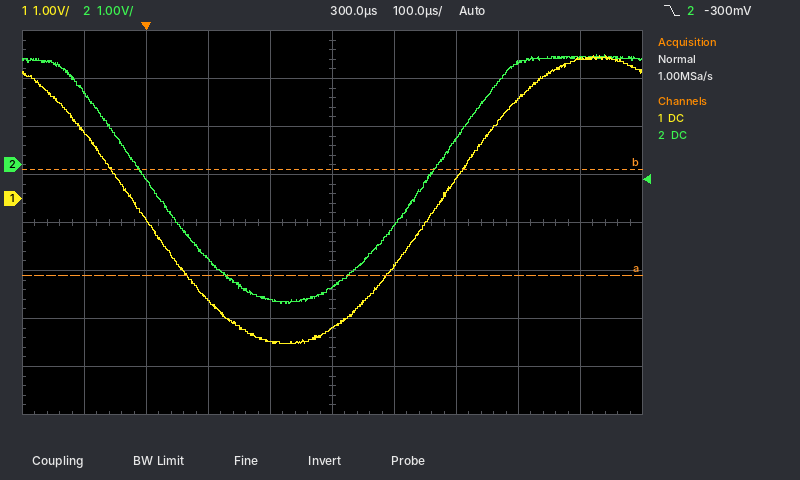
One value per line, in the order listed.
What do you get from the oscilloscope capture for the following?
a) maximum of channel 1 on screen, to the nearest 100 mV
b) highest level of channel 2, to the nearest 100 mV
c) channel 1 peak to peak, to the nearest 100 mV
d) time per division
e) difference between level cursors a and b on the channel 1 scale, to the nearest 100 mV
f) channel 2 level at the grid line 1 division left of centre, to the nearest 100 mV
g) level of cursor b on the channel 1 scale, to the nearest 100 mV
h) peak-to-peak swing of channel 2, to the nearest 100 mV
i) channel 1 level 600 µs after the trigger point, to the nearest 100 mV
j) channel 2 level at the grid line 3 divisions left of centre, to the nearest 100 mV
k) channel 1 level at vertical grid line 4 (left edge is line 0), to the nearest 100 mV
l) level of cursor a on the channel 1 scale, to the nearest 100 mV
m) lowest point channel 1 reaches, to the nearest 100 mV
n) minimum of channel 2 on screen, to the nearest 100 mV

3.0 V
2.3 V
6.0 V
100 µs
2.2 V
-2.8 V
600 mV
5.2 V
2.1 V
-300 mV
-3.0 V
-1.6 V
-3.0 V
-2.9 V
